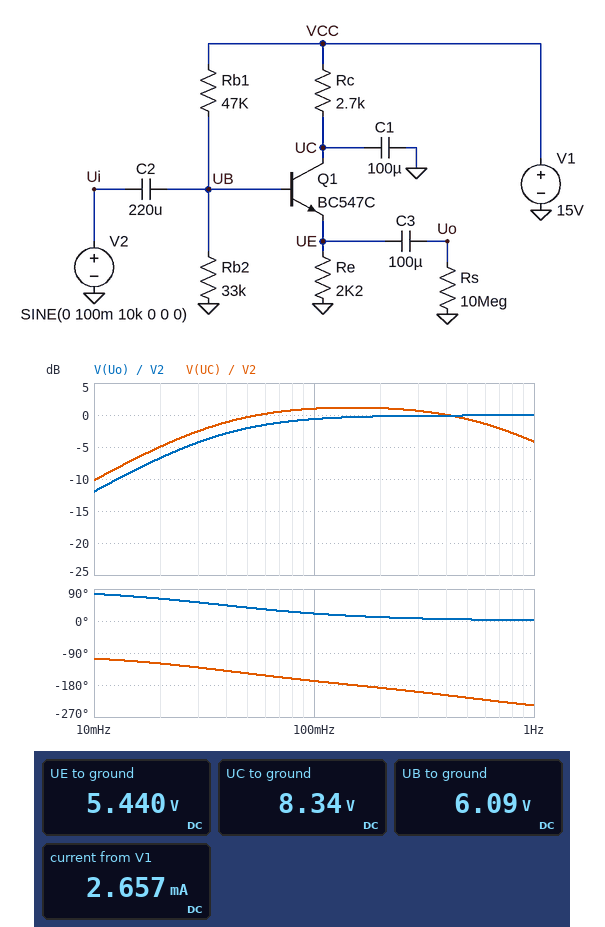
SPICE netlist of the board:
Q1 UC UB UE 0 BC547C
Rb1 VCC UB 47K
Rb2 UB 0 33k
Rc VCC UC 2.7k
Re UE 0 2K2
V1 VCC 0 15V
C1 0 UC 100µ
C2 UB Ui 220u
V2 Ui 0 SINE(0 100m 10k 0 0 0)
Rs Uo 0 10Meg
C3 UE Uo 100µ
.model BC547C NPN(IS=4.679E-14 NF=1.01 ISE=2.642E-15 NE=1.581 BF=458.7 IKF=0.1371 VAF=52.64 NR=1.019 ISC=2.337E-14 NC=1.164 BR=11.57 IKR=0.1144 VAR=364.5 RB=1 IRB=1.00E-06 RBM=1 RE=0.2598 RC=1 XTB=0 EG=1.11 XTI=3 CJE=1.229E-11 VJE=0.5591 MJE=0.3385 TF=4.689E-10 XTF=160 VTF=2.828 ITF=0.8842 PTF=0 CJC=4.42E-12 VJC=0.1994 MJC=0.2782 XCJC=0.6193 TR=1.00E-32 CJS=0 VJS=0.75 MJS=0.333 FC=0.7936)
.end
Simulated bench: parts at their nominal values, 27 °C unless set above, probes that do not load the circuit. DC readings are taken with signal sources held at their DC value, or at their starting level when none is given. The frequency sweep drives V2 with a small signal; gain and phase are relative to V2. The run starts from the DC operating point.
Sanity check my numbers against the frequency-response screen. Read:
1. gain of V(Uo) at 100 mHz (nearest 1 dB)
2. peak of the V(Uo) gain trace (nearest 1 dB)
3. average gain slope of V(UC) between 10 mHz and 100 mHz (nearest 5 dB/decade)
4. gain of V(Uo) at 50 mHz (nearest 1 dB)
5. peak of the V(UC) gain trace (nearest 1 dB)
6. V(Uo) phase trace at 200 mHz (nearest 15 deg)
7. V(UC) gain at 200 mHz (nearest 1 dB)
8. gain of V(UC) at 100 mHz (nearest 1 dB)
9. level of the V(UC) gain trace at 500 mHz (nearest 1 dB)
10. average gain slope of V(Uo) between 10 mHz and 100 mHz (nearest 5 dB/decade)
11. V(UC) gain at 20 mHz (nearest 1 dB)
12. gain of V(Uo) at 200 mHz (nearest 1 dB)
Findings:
-1 dB
0 dB
10 dB/decade
-2 dB
1 dB
15 deg
1 dB
1 dB
-1 dB
10 dB/decade
-5 dB
0 dB
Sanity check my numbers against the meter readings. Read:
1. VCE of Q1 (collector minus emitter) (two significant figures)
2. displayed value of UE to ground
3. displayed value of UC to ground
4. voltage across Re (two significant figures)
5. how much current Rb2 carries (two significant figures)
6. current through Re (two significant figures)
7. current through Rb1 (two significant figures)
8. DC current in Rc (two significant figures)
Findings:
2.9 V
5.440 V
8.34 V
5.4 V
180 µA
2.5 mA
190 µA
2.5 mA
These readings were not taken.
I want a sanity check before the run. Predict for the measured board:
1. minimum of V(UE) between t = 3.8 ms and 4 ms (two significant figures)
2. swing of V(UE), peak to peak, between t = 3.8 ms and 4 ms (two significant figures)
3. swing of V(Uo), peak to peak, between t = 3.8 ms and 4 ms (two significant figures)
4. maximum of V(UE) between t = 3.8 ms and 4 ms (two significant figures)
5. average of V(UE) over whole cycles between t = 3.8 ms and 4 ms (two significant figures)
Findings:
5.3 V
200 mV
200 mV
5.5 V
5.4 V
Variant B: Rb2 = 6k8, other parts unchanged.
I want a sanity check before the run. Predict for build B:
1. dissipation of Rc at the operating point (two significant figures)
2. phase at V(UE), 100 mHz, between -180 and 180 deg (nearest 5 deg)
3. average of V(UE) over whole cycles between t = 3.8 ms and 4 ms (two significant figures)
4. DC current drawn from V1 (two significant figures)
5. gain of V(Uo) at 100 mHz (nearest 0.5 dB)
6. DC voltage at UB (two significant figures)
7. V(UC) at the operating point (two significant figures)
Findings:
920 µW
50 deg
1.3 V
860 µA
-4.0 dB
1.9 V
13 V
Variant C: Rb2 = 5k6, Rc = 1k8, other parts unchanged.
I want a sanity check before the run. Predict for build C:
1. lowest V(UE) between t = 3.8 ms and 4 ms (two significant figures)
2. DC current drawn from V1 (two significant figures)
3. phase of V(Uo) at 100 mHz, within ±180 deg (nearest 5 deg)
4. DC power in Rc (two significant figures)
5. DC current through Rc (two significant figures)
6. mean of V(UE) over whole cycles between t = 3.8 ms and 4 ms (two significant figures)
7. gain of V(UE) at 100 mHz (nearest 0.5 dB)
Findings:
900 mV
740 µA
55 deg
370 µW
450 µA
1.0 V
-5.0 dB
